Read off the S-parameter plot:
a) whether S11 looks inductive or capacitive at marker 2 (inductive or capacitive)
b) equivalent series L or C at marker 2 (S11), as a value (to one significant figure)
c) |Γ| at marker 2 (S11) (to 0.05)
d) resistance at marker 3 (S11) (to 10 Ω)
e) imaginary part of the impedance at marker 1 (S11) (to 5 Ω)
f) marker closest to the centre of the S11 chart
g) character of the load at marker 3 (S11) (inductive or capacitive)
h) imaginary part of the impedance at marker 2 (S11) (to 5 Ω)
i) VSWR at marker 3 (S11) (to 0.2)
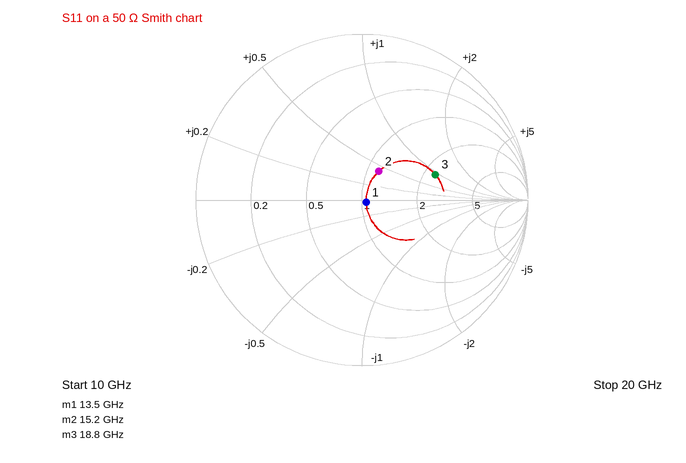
inductive
200 pH
0.20
120 Ω
0 Ω
marker 1
inductive
+20 Ω
2.8
